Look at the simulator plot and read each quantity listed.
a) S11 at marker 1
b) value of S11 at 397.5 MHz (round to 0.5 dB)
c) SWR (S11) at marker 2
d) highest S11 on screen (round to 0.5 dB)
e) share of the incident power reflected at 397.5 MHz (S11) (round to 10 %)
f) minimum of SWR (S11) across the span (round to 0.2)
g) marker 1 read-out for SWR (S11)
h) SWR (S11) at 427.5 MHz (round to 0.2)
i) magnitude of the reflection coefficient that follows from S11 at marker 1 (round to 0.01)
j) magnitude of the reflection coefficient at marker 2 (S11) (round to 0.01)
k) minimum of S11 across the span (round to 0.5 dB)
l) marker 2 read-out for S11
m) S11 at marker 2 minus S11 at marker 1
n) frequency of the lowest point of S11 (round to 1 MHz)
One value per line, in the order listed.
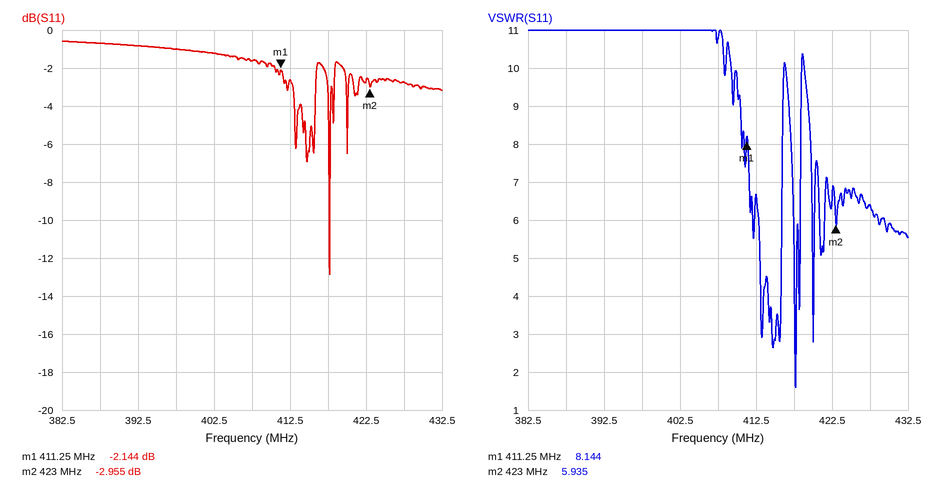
-2.144 dB
-1.0 dB
5.935
-0.5 dB
80 %
1.6
8.144
6.4
0.78
0.71
-13.0 dB
-2.955 dB
-0.811 dB
418 MHz
